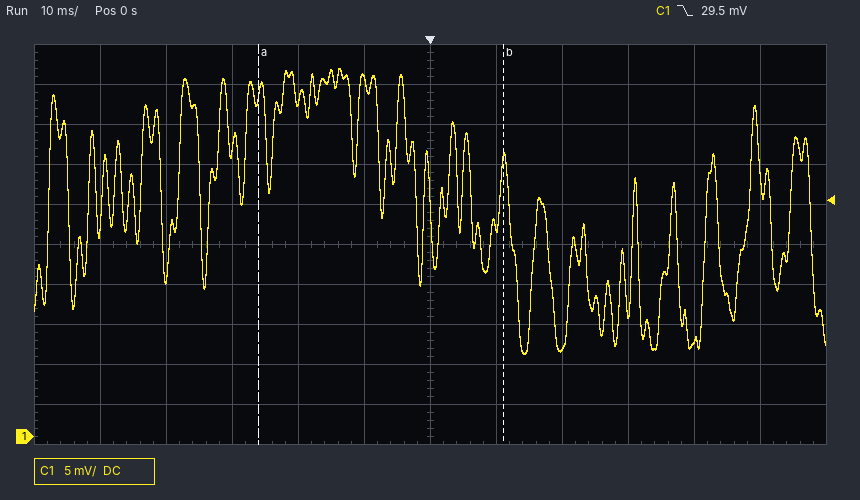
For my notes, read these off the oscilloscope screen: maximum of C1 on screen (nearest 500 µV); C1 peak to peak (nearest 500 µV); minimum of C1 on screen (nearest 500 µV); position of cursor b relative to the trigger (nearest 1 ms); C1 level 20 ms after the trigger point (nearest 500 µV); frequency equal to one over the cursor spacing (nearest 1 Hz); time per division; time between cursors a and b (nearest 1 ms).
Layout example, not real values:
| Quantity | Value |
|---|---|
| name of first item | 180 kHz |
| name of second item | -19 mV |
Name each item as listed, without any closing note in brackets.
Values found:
| Quantity | Value |
|---|---|
| maximum of C1 on screen | 46.0 mV |
| C1 peak to peak | 35.5 mV |
| minimum of C1 on screen | 10.5 mV |
| position of cursor b relative to the trigger | +11 ms |
| C1 level 20 ms after the trigger point | 11.0 mV |
| frequency equal to one over the cursor spacing | 27 Hz |
| time per division | 10 ms |
| time between cursors a and b | 37 ms |
